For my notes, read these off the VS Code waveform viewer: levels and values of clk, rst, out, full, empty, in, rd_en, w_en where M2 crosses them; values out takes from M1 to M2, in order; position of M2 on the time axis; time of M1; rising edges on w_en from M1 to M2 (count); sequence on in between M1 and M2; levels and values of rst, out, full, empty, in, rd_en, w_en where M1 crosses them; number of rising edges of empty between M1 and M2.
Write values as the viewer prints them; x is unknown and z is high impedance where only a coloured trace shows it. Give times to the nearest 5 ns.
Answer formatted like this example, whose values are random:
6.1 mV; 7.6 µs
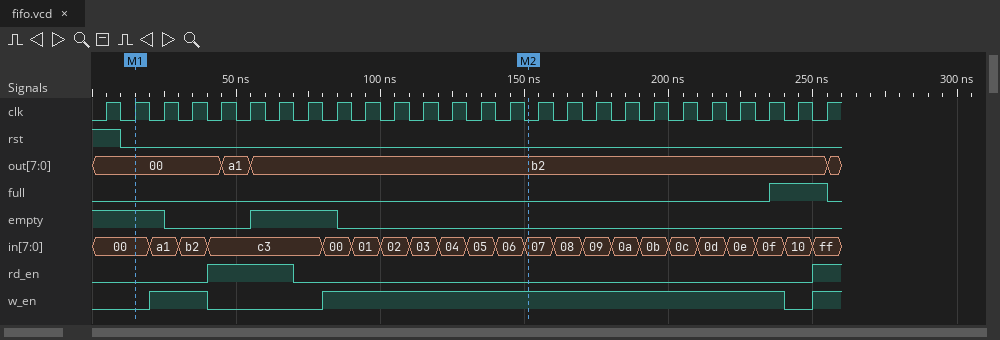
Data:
clk=0, rst=0, out=b2, full=0, empty=0, in=07, rd_en=0, w_en=1; 00, a1, b2; 150 ns; 15 ns; 2; 00, a1, b2, c3, 00, 01, 02, 03, 04, 05, 06, 07; rst=0, out=00, full=0, empty=1, in=00, rd_en=0, w_en=0; 1
